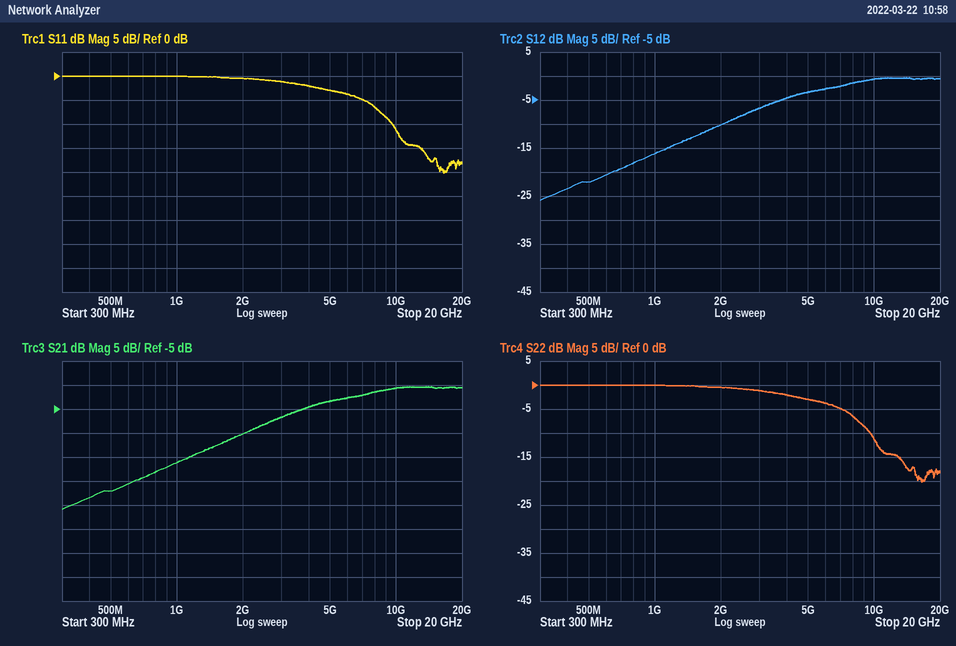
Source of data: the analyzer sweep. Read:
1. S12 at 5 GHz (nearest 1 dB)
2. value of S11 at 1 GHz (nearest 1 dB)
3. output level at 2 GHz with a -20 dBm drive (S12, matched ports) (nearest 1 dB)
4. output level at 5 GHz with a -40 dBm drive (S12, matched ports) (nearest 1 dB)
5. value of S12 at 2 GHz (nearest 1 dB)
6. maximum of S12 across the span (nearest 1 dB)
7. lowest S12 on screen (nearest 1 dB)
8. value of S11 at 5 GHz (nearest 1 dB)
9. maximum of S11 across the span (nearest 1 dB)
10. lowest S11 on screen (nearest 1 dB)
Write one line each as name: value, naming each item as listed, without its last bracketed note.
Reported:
S12 at 5 GHz: -3 dB
value of S11 at 1 GHz: 0 dB
output level at 2 GHz with a -20 dBm drive (S12, matched ports): -30 dBm
output level at 5 GHz with a -40 dBm drive (S12, matched ports): -43 dBm
value of S12 at 2 GHz: -10 dB
maximum of S12 across the span: 0 dB
lowest S12 on screen: -26 dB
value of S11 at 5 GHz: -3 dB
maximum of S11 across the span: 0 dB
lowest S11 on screen: -20 dB
